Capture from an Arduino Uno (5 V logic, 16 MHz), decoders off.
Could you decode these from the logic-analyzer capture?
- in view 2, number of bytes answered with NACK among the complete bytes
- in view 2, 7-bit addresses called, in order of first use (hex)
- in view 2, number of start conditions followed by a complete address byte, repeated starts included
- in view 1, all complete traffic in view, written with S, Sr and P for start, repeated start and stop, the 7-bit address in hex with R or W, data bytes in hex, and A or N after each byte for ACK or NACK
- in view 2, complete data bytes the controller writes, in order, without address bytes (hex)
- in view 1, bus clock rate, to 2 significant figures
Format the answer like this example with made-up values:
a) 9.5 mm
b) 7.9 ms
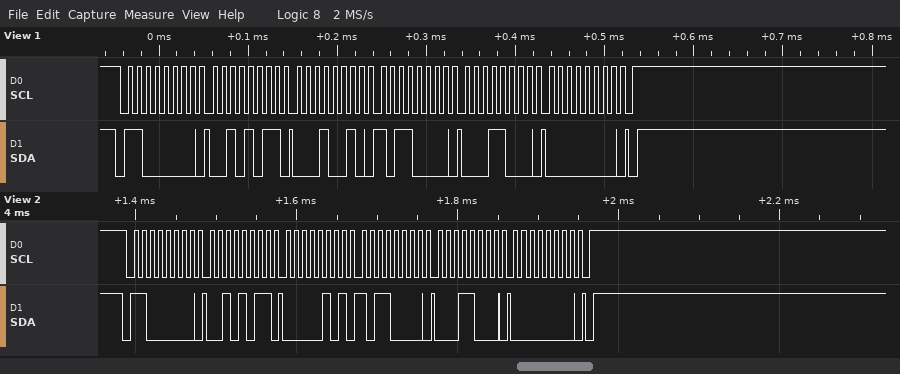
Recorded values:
a) 0
b) 0x60
c) 1
d) S 60W A 2B A 12 A B0 A 18 A 00 A P
e) 2B 05 B0 18 00
f) 100 kHz
